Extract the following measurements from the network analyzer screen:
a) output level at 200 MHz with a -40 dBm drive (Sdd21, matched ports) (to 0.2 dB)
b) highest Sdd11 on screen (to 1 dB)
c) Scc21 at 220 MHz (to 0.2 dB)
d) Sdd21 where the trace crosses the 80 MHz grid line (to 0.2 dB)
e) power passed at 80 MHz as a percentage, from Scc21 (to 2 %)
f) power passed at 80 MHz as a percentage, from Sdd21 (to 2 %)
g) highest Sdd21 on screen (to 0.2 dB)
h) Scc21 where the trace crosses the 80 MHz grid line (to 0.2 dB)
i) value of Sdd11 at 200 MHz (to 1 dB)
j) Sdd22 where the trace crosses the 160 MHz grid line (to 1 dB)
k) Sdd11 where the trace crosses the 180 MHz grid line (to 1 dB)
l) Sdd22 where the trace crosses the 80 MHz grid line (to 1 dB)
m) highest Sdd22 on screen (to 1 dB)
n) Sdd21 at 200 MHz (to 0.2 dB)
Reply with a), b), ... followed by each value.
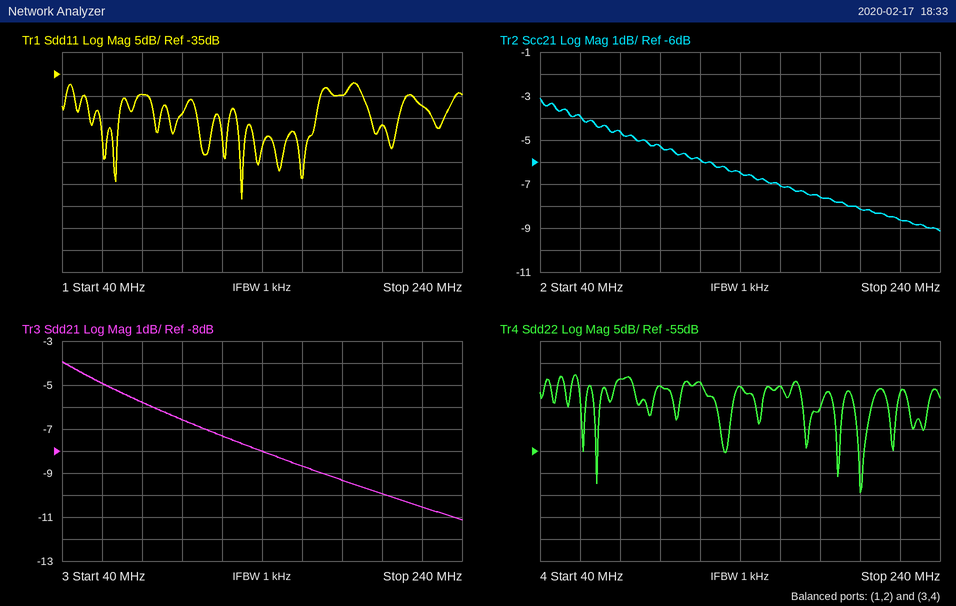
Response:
a) -50.0 dBm
b) -37 dB
c) -8.6 dB
d) -5.8 dB
e) 34 %
f) 26 %
g) -4.0 dB
h) -4.6 dB
i) -47 dB
j) -40 dB
k) -40 dB
l) -39 dB
m) -38 dB
n) -10.0 dB
